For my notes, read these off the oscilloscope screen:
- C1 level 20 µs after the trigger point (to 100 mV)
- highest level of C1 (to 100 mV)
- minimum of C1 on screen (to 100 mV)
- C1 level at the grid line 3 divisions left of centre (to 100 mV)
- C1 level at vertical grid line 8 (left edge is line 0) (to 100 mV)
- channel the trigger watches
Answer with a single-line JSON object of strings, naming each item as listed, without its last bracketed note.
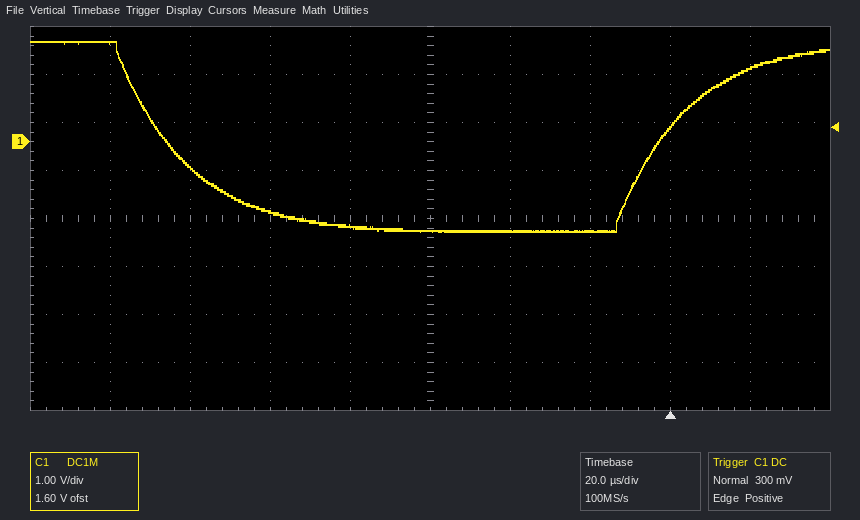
{"C1 level 20 µs after the trigger point": "1.5 V", "highest level of C1": "2.1 V", "minimum of C1 on screen": "-1.9 V", "C1 level at the grid line 3 divisions left of centre": "-500 mV", "C1 level at vertical grid line 8 (left edge is line 0)": "300 mV", "channel the trigger watches": "C1"}
